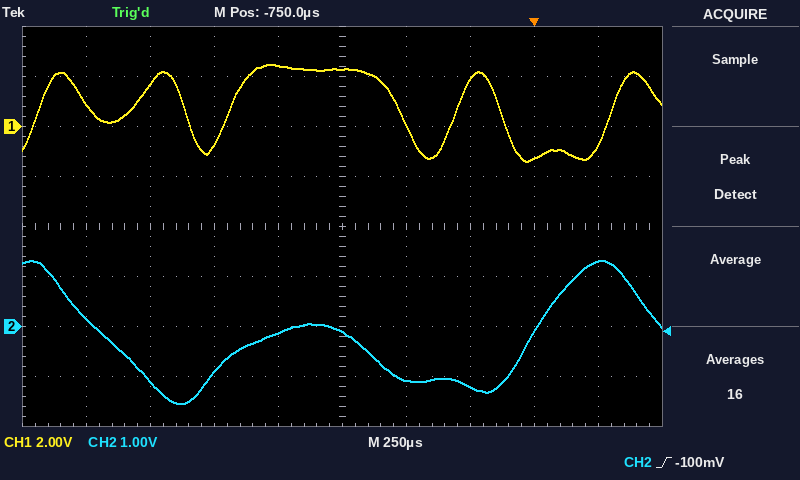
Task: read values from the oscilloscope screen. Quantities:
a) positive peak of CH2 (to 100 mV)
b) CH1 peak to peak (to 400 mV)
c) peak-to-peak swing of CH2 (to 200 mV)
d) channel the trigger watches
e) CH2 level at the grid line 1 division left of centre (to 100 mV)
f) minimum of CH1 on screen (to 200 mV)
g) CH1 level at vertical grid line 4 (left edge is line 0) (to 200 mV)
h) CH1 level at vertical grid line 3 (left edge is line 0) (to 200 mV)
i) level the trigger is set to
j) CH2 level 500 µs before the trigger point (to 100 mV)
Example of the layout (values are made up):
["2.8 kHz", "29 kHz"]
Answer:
["1.3 V", "4.0 V", "2.8 V", "CH2", "-100 mV", "-1.4 V", "2.4 V", "-800 mV", "-100 mV", "-1.1 V"]
